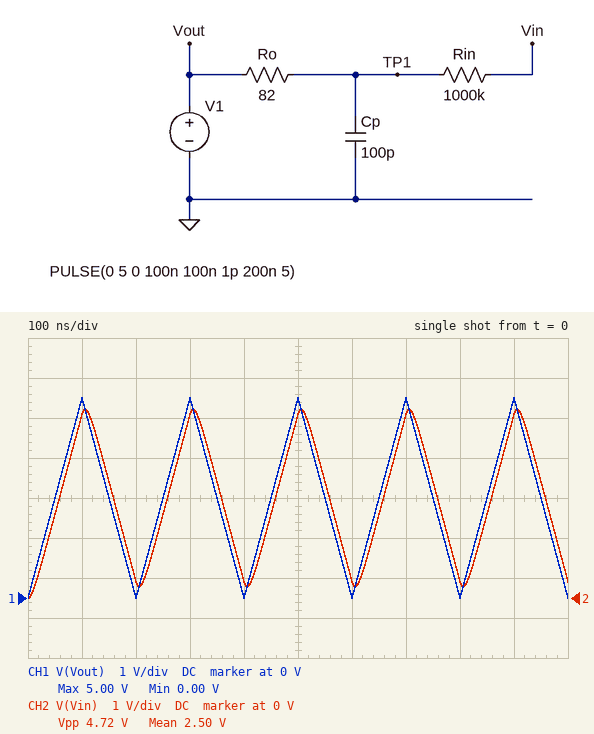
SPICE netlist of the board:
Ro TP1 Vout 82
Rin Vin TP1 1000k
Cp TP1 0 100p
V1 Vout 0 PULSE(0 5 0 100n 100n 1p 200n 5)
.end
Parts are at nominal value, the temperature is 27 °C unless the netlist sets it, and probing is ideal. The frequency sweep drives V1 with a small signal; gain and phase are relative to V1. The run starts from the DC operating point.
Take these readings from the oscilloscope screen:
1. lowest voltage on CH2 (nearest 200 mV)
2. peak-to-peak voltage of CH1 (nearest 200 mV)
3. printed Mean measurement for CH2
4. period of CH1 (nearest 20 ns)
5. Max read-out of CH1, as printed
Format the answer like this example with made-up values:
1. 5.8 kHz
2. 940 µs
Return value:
1. 0 V
2. 5.0 V
3. 2.50 V
4. 200 ns
5. 5.00 V
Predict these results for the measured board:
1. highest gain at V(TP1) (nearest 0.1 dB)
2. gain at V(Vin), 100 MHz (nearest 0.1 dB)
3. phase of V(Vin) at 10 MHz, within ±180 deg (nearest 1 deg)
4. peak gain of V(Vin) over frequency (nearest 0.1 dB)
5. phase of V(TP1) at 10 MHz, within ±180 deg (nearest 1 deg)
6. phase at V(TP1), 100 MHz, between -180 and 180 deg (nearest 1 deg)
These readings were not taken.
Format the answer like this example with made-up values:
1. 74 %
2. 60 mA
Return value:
1. 0 dB
2. -14.4 dB
3. -27 deg
4. 0 dB
5. -27 deg
6. -79 deg
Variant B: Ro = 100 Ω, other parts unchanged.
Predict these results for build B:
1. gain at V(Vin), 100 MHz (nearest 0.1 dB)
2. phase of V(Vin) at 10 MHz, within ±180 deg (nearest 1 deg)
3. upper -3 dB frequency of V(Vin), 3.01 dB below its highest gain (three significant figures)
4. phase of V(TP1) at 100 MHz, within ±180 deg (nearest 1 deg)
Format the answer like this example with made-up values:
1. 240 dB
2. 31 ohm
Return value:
1. -16.1 dB
2. -32 deg
3. 15.9 MHz
4. -81 deg
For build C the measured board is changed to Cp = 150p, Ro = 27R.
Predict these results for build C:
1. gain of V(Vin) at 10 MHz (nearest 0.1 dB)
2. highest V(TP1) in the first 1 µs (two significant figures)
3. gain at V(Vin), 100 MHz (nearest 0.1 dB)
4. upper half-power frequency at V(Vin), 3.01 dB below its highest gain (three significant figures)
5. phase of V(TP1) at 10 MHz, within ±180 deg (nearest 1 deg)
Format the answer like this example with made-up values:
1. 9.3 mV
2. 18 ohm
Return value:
1. -0.3 dB
2. 4.9 V
3. -8.7 dB
4. 39.3 MHz
5. -14 deg
